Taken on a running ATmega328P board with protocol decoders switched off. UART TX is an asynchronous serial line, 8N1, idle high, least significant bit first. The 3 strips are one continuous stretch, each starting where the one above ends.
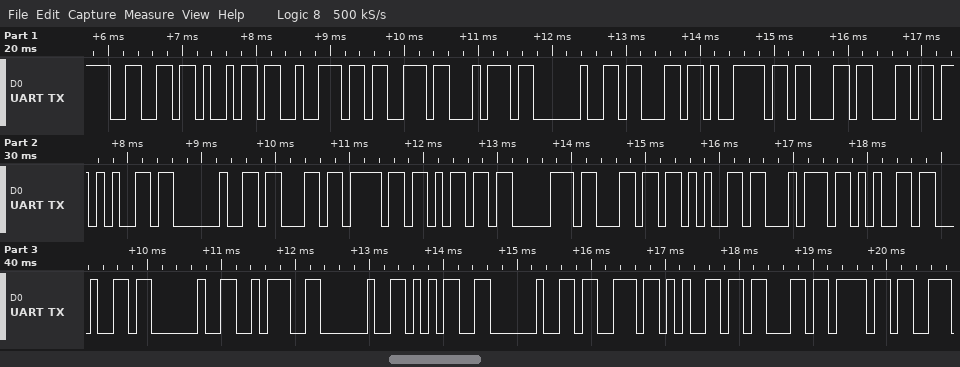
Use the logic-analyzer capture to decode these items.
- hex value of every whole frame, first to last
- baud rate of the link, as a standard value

66 69 72 73 74 20 63 79 63 6C 65 20 63 6F 6D 70 6C 65 74 65 64 20 3A 20 35 20 73 65 63 6F
9600 baud
